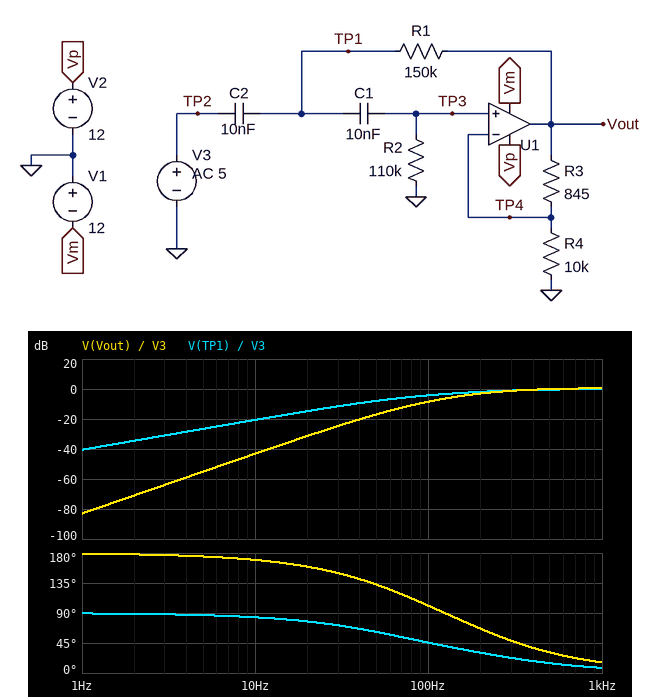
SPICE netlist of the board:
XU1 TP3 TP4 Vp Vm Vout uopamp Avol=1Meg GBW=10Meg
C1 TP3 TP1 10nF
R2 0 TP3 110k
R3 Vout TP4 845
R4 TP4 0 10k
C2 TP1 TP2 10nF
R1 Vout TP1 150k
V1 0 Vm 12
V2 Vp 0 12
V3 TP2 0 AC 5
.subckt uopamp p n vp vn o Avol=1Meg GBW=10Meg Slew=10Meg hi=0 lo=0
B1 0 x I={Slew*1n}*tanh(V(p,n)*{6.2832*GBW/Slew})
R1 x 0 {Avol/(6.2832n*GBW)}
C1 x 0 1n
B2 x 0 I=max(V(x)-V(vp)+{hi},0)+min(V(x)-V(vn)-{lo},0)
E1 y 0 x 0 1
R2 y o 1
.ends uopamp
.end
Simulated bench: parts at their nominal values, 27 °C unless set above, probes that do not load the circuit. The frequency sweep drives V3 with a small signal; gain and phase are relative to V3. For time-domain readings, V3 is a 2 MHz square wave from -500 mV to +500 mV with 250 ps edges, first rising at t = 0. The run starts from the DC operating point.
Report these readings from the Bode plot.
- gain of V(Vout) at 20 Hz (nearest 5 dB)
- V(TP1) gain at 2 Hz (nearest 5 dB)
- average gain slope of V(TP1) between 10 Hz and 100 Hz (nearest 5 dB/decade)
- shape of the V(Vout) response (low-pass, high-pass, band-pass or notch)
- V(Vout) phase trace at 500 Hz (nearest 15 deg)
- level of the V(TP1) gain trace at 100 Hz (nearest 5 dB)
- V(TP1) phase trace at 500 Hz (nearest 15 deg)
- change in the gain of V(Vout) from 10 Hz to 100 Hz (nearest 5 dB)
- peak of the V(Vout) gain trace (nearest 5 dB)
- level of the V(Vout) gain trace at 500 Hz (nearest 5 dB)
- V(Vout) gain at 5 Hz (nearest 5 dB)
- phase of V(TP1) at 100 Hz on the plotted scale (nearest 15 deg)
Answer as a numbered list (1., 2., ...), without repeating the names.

1. -30 dB
2. -35 dB
3. 15 dB/decade
4. high-pass
5. 30 deg
6. -5 dB
7. 15 deg
8. 35 dB
9. 0 dB
10. 0 dB
11. -55 dB
12. 45 deg
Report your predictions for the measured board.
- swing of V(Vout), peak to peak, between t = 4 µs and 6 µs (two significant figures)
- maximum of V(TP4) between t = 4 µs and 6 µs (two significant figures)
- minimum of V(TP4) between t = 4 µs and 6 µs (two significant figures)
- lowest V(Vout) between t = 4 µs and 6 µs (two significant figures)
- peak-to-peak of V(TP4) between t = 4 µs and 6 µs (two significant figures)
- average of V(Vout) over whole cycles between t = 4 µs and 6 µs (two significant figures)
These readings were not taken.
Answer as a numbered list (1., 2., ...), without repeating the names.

1. 1.1 V
2. 1.0 V
3. -5.2 mV
4. -5.7 mV
5. 1.0 V
6. 540 mV
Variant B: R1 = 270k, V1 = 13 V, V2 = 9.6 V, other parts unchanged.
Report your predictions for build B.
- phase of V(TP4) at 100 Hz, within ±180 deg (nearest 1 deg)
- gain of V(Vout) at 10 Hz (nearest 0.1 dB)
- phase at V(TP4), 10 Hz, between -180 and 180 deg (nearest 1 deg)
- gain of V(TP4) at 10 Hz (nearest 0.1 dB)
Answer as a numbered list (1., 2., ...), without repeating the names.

1. 87 deg
2. -38.3 dB
3. 161 deg
4. -39.0 dB
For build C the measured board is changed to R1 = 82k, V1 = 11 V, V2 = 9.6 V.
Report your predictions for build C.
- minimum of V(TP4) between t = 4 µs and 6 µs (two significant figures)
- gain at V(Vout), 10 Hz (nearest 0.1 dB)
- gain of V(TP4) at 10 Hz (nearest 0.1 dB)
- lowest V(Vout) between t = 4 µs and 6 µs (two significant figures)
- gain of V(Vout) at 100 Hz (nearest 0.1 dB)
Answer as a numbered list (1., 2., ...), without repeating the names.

1. -5.1 mV
2. -48.3 dB
3. -49.0 dB
4. -5.5 mV
5. -9.6 dB
